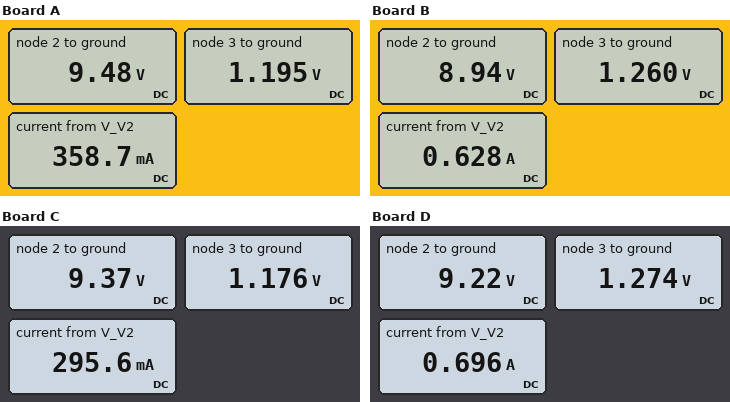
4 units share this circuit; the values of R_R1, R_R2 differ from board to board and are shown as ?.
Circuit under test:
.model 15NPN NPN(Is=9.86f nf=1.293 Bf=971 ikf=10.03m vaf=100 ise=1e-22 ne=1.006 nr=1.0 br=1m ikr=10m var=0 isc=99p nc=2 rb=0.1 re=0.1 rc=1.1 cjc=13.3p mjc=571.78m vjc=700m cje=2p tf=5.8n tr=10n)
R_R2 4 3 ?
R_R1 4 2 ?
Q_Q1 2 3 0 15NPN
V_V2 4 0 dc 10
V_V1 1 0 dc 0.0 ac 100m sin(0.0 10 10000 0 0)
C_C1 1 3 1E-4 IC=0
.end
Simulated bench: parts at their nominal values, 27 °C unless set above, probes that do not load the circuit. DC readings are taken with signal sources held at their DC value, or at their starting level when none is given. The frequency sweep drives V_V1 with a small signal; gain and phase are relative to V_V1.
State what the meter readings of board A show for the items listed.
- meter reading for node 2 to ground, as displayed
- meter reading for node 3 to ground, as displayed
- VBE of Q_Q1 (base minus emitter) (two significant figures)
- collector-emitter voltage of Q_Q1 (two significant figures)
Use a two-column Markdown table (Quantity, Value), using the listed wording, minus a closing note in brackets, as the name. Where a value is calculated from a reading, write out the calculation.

| Quantity | Value |
|---|---|
| meter reading for node 2 to ground, as displayed | 9.48 V |
| meter reading for node 3 to ground, as displayed | 1.195 V |
| VBE of Q_Q1 (base minus emitter) | 1.195 V = 1.2 V |
| collector-emitter voltage of Q_Q1 | 9.48 V = 9.5 V |
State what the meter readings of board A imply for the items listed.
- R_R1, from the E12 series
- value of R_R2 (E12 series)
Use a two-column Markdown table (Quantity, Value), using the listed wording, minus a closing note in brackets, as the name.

| Quantity | Value |
|---|---|
| R_R1, from the E12 series | 1.5 Ω |
| value of R_R2 | 680 Ω |
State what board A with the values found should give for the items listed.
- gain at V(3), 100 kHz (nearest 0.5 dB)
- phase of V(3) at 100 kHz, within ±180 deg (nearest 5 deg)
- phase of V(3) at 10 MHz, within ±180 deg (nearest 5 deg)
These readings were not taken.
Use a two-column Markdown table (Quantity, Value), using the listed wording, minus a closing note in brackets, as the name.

| Quantity | Value |
|---|---|
| gain at V(3), 100 kHz | 0 dB |
| phase of V(3) at 100 kHz, within ±180 deg | 0 deg |
| phase of V(3) at 10 MHz, within ±180 deg | 0 deg |
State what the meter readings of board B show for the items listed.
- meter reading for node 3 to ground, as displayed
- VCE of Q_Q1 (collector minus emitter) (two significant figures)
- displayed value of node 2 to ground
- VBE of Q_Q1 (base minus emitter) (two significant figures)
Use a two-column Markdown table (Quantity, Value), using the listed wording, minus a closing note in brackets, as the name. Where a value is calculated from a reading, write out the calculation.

| Quantity | Value |
|---|---|
| meter reading for node 3 to ground, as displayed | 1.260 V |
| VCE of Q_Q1 (collector minus emitter) | 8.94 V = 8.9 V |
| displayed value of node 2 to ground | 8.94 V |
| VBE of Q_Q1 (base minus emitter) | 1.26 V = 1.3 V |
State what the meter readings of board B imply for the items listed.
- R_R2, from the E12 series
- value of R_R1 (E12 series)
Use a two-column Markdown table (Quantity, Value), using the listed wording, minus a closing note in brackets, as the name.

| Quantity | Value |
|---|---|
| R_R2, from the E12 series | 220 Ω |
| value of R_R1 | 1.8 Ω |
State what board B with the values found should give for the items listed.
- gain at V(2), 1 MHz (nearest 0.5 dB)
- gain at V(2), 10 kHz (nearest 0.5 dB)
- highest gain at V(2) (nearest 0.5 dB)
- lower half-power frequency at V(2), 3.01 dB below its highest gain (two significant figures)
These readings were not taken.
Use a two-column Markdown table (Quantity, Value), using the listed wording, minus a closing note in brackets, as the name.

| Quantity | Value |
|---|---|
| gain at V(2), 1 MHz | 17.5 dB |
| gain at V(2), 10 kHz | 17.5 dB |
| highest gain at V(2) | 17.5 dB |
| lower half-power frequency at V(2), 3.01 dB below its highest gain | 950 Hz |
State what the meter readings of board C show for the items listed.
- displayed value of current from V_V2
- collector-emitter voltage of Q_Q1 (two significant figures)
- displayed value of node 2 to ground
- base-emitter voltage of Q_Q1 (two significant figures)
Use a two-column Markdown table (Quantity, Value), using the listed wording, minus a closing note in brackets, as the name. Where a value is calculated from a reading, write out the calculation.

| Quantity | Value |
|---|---|
| displayed value of current from V_V2 | 295.6 mA |
| collector-emitter voltage of Q_Q1 | 9.37 V = 9.4 V |
| displayed value of node 2 to ground | 9.37 V |
| base-emitter voltage of Q_Q1 | 1.176 V = 1.2 V |
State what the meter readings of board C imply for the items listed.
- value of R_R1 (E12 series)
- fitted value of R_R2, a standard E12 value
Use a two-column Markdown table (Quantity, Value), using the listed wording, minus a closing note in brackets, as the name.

| Quantity | Value |
|---|---|
| value of R_R1 | 2.2 Ω |
| fitted value of R_R2, a standard E12 value | 1 kΩ |
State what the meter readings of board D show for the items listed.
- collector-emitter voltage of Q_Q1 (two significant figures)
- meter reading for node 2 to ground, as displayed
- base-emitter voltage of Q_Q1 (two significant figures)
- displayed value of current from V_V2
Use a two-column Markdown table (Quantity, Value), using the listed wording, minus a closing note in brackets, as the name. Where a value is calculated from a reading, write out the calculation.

| Quantity | Value |
|---|---|
| collector-emitter voltage of Q_Q1 | 9.22 V = 9.2 V |
| meter reading for node 2 to ground, as displayed | 9.22 V |
| base-emitter voltage of Q_Q1 | 1.274 V = 1.3 V |
| displayed value of current from V_V2 | 0.696 A |
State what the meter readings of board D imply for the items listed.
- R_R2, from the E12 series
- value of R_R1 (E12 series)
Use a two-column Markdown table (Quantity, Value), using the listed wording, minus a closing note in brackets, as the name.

| Quantity | Value |
|---|---|
| R_R2, from the E12 series | 180 Ω |
| value of R_R1 | 1.2 Ω |
